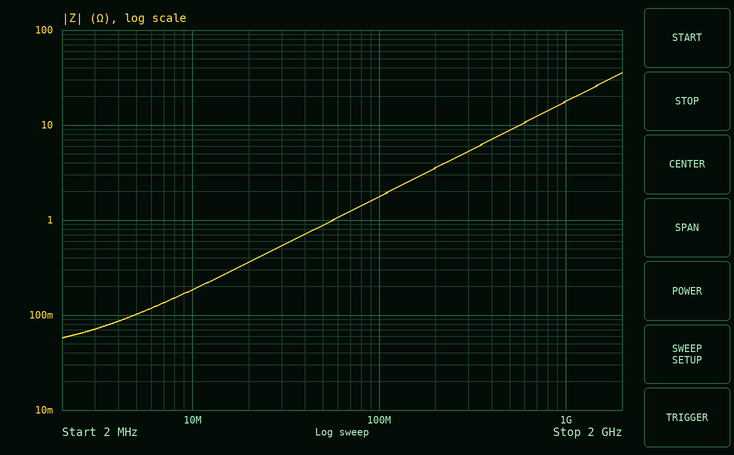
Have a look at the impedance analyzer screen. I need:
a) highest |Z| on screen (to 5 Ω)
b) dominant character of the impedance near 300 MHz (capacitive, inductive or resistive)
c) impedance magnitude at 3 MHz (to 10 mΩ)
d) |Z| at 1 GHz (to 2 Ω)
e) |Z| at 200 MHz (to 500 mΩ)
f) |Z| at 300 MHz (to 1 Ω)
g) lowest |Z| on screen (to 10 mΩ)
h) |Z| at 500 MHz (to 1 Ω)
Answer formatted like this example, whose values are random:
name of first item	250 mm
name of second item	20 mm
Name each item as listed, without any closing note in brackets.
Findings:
highest |Z| on screen	35 Ω
dominant character of the impedance near 300 MHz	inductive
impedance magnitude at 3 MHz	70 mΩ
|Z| at 1 GHz	18 Ω
|Z| at 200 MHz	3.5 Ω
|Z| at 300 MHz	5 Ω
lowest |Z| on screen	60 mΩ
|Z| at 500 MHz	9 Ω
